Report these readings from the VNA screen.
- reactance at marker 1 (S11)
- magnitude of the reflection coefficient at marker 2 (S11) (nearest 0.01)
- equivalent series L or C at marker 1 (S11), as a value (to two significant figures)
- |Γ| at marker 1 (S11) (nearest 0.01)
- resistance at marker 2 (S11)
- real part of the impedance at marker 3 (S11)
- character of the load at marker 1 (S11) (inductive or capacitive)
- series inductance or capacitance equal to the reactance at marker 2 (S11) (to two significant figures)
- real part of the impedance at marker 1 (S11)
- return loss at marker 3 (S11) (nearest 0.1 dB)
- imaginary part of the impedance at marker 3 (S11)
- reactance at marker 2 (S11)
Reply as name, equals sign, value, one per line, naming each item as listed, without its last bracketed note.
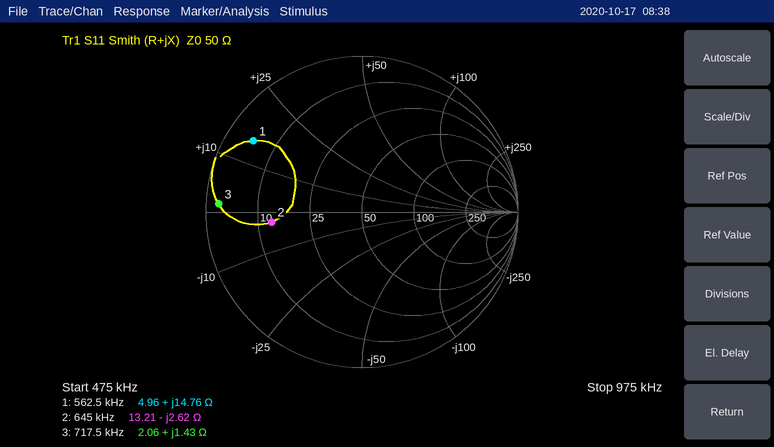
reactance at marker 1 = +14.76 Ω
magnitude of the reflection coefficient at marker 2 (S11) = 0.58
equivalent series L or C at marker 1 (S11), as a value = 4.2 µH
|Γ| at marker 1 (S11) = 0.83
resistance at marker 2 = 13.21 Ω
real part of the impedance at marker 3 = 2.06 Ω
character of the load at marker 1 (S11) = inductive
series inductance or capacitance equal to the reactance at marker 2 (S11) = 94 nF
real part of the impedance at marker 1 = 4.96 Ω
return loss at marker 3 (S11) = 0.7 dB
imaginary part of the impedance at marker 3 = +1.43 Ω
reactance at marker 2 = -2.62 Ω
